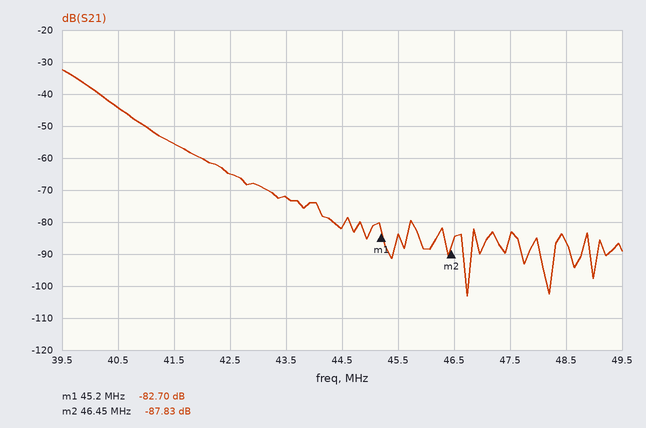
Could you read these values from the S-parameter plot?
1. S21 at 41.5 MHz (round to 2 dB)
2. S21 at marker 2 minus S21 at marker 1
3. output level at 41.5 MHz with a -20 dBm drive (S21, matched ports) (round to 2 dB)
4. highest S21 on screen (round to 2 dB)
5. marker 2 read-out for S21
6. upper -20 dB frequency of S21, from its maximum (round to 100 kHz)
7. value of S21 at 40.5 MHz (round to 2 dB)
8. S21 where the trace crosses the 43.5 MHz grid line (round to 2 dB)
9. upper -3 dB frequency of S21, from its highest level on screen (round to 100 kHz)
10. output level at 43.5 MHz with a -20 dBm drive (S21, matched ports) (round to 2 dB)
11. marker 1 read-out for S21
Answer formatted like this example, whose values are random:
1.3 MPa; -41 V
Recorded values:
-56 dB; -5.13 dB; -76 dBm; -32 dB; -87.83 dB; 41.2 MHz; -44 dB; -72 dB; 39.8 MHz; -92 dBm; -82.70 dB
